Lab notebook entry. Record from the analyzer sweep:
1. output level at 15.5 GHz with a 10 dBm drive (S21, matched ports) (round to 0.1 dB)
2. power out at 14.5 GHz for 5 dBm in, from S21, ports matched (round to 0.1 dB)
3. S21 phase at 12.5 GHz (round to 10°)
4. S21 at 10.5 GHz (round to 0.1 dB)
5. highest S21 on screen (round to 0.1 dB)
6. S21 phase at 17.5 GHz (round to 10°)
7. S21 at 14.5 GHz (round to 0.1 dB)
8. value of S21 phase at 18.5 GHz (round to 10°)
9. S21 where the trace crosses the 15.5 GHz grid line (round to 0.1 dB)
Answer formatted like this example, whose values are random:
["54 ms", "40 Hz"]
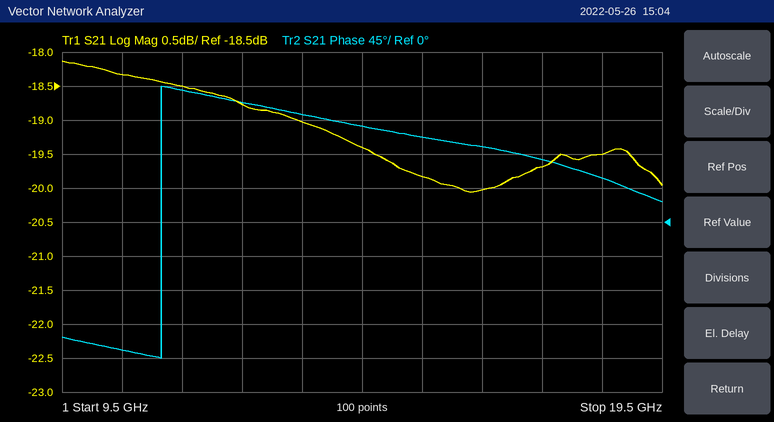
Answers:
["-9.8 dBm", "-14.4 dBm", "160°", "-18.3 dB", "-18.1 dB", "80°", "-19.4 dB", "60°", "-19.8 dB"]
